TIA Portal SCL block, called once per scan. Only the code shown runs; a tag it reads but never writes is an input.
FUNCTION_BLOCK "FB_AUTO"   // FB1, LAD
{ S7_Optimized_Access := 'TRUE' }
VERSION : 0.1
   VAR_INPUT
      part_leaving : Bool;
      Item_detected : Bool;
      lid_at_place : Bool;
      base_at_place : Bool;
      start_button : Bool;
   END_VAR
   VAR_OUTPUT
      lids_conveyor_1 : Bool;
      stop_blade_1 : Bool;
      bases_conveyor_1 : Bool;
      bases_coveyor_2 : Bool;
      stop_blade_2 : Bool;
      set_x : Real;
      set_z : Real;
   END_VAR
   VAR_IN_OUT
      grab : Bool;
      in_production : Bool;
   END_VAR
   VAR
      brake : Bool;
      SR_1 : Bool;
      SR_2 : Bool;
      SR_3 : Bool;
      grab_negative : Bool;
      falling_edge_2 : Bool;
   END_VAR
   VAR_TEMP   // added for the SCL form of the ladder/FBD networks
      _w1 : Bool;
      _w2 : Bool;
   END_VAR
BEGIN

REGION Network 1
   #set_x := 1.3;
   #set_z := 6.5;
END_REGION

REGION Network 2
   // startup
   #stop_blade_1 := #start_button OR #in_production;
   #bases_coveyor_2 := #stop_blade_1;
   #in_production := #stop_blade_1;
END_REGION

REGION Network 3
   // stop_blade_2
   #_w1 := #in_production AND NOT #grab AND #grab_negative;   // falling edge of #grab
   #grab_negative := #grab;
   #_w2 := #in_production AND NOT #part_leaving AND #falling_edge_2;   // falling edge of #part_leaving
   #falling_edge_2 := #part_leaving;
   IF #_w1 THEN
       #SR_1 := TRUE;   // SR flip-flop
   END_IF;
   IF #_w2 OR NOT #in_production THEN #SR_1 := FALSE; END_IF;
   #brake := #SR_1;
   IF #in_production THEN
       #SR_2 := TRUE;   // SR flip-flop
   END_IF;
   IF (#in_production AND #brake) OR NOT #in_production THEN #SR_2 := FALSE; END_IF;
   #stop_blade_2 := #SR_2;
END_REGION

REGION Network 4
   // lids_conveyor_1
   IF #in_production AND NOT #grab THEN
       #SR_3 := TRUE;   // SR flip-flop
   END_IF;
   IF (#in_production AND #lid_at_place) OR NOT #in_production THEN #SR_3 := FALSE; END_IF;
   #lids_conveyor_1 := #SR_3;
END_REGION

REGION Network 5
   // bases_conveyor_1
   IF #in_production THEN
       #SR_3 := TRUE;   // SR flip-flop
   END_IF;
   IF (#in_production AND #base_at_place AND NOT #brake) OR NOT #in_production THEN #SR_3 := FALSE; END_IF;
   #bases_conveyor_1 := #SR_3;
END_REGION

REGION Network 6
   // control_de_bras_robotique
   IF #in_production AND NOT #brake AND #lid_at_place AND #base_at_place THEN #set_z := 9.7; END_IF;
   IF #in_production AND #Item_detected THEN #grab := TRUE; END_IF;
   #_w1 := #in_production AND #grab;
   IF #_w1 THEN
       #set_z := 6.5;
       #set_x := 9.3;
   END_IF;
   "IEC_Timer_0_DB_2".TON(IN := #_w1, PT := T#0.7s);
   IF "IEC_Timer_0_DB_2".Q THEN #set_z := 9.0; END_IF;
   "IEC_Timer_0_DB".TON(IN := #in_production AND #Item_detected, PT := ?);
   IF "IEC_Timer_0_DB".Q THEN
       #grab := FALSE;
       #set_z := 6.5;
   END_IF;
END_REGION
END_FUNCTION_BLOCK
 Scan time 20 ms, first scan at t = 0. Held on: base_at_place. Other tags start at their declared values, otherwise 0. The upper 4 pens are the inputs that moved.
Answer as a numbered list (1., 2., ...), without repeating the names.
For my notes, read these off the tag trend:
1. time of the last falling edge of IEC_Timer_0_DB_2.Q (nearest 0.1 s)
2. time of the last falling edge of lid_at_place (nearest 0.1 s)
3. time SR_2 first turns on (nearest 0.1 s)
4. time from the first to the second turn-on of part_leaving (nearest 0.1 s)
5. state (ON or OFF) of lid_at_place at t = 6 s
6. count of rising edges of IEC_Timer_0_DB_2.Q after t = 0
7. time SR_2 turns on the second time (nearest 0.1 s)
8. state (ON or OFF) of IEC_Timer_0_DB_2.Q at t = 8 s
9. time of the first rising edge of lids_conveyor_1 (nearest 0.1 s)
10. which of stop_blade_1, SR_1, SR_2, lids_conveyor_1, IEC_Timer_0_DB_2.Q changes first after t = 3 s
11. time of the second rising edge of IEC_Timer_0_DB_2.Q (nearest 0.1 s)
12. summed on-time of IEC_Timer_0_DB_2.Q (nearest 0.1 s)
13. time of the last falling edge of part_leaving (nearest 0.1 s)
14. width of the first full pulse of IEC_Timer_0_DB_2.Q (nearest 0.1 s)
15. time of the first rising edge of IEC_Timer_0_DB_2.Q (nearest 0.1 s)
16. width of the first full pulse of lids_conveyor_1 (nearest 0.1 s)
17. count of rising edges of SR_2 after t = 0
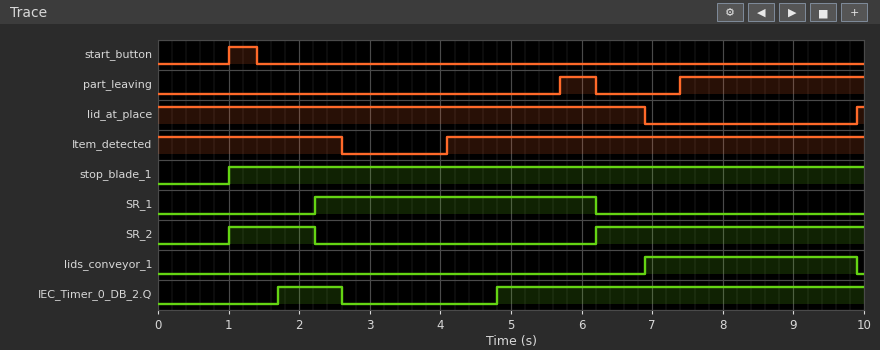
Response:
1. 2.6 s
2. 6.9 s
3. 1.0 s
4. 1.7 s
5. ON
6. 2
7. 6.2 s
8. ON
9. 6.9 s
10. IEC_Timer_0_DB_2.Q
11. 4.8 s
12. 6.1 s
13. 6.2 s
14. 0.9 s
15. 1.7 s
16. 3.0 s
17. 2
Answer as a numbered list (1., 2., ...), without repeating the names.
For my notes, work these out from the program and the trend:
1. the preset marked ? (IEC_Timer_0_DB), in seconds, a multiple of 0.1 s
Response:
1. 1.2 s
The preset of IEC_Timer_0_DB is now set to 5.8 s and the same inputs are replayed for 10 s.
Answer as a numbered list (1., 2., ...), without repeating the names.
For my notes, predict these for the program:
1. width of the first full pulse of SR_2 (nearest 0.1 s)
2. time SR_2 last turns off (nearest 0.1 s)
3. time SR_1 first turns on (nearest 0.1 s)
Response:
1. 8.9 s
2. 9.9 s
3. 9.9 s
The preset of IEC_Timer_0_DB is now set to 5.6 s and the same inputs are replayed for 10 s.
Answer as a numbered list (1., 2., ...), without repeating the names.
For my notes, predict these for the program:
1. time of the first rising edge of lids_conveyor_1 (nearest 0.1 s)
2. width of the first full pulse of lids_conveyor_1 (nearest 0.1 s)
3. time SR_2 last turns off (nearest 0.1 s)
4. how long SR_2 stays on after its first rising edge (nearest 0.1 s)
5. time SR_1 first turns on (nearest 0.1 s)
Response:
1. 9.7 s
2. 0.2 s
3. 9.7 s
4. 8.7 s
5. 9.7 s
